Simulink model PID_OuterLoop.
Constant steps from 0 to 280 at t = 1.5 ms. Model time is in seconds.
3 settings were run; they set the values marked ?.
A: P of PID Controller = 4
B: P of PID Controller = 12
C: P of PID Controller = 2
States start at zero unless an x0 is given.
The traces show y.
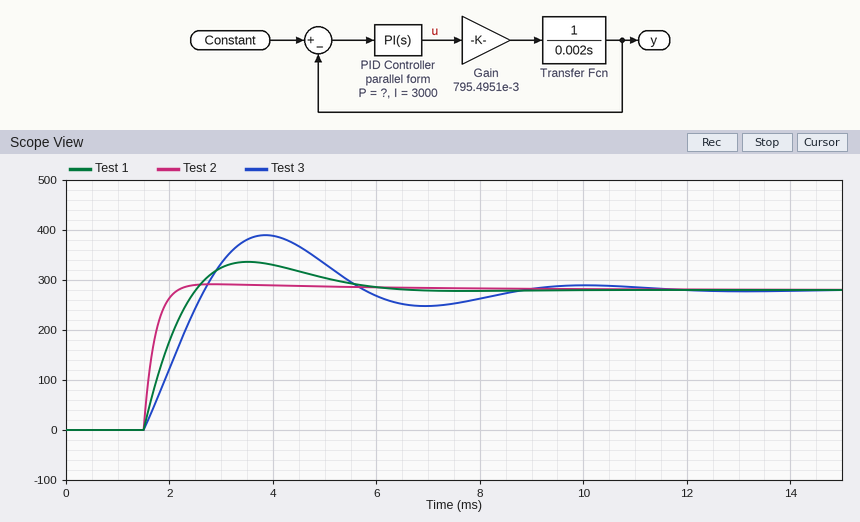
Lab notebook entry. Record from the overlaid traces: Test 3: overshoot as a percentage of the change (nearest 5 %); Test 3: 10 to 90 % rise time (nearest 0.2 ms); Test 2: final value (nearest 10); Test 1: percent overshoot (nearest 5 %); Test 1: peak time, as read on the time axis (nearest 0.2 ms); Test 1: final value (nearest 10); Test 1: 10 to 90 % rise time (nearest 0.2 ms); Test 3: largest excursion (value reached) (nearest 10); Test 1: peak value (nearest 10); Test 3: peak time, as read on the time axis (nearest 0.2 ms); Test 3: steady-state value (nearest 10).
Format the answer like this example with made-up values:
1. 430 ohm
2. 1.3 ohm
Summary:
1. 40 %
2. 1.0 ms
3. 280
4. 20 %
5. 3.6 ms
6. 280
7. 0.8 ms
8. 390
9. 340
10. 3.8 ms
11. 280
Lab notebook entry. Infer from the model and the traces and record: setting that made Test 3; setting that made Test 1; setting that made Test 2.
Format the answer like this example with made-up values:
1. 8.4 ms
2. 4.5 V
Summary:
1. C
2. A
3. B
